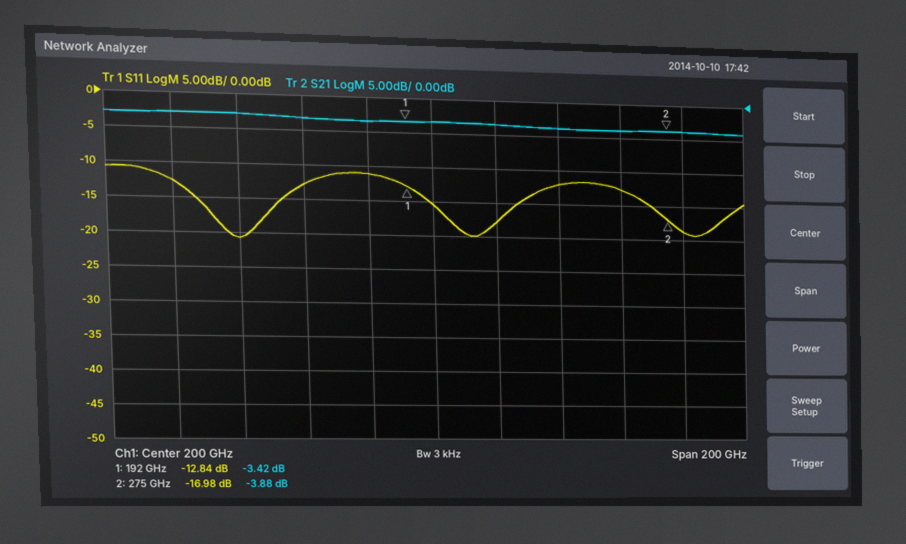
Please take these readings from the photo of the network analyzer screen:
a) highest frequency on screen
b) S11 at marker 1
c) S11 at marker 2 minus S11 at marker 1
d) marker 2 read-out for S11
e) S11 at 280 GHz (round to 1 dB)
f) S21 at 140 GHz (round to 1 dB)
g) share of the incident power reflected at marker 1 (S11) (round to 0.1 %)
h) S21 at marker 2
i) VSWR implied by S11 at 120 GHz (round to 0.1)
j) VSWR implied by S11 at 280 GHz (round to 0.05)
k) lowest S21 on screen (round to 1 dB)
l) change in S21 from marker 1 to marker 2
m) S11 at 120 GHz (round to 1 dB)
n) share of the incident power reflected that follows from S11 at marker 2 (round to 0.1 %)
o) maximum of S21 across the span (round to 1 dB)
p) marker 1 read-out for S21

300 GHz
-12.84 dB
-4.14 dB
-16.98 dB
-19 dB
-3 dB
5.2 %
-3.88 dB
1.6
1.25
-4 dB
-0.46 dB
-13 dB
2.0 %
-3 dB
-3.42 dB
